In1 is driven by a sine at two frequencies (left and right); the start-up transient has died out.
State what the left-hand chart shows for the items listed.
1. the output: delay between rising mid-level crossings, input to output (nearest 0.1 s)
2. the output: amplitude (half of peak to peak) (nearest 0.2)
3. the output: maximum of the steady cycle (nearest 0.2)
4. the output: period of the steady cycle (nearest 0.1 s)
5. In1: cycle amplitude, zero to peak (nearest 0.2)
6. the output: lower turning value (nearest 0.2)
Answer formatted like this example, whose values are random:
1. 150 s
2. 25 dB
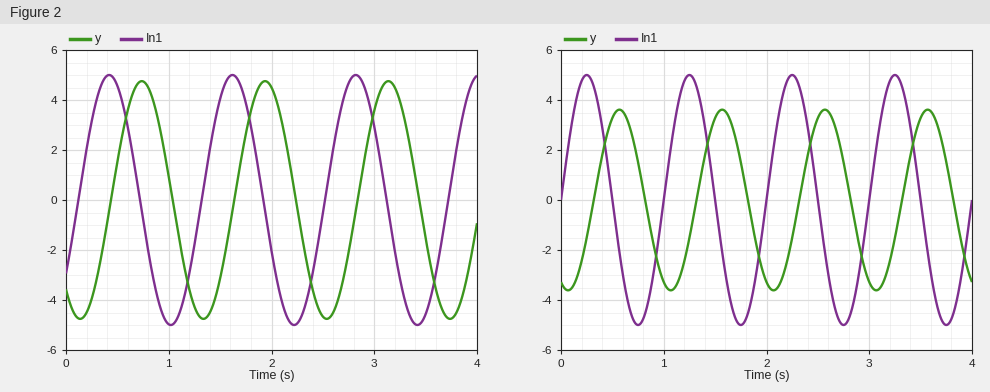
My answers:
1. 0.3 s
2. 4.8
3. 4.8
4. 1.2 s
5. 5.0
6. -4.8
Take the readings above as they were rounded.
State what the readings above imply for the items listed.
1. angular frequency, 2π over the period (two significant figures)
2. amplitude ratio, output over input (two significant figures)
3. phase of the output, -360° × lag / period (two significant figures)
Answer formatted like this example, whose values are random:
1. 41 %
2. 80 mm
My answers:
1. 5.2 rad/s
2. 0.96
3. -90°
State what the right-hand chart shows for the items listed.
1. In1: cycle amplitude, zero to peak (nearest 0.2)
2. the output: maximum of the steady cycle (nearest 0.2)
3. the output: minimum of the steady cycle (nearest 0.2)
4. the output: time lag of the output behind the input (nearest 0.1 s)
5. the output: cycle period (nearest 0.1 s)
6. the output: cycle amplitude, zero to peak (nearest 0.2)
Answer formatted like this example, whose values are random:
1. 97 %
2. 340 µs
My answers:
1. 5.0
2. 3.6
3. -3.6
4. 0.3 s
5. 1.0 s
6. 3.6
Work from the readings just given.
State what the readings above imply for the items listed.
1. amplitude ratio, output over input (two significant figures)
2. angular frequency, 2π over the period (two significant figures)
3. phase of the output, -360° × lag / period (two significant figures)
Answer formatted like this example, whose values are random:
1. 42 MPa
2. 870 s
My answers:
1. 0.72
2. 6.3 rad/s
3. -110°
